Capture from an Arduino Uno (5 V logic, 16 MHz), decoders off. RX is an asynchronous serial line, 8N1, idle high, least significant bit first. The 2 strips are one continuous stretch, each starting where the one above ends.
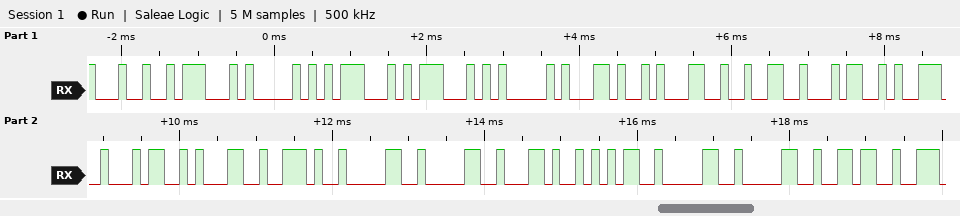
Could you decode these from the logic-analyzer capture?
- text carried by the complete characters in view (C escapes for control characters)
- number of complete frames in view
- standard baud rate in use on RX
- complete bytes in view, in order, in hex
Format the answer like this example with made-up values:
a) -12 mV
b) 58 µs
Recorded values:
a) "$GPGGA,124941.00,5006"
b) 21
c) 9600 baud
d) 24 47 50 47 47 41 2C 31 32 34 39 34 31 2E 30 30 2C 35 30 30 36
